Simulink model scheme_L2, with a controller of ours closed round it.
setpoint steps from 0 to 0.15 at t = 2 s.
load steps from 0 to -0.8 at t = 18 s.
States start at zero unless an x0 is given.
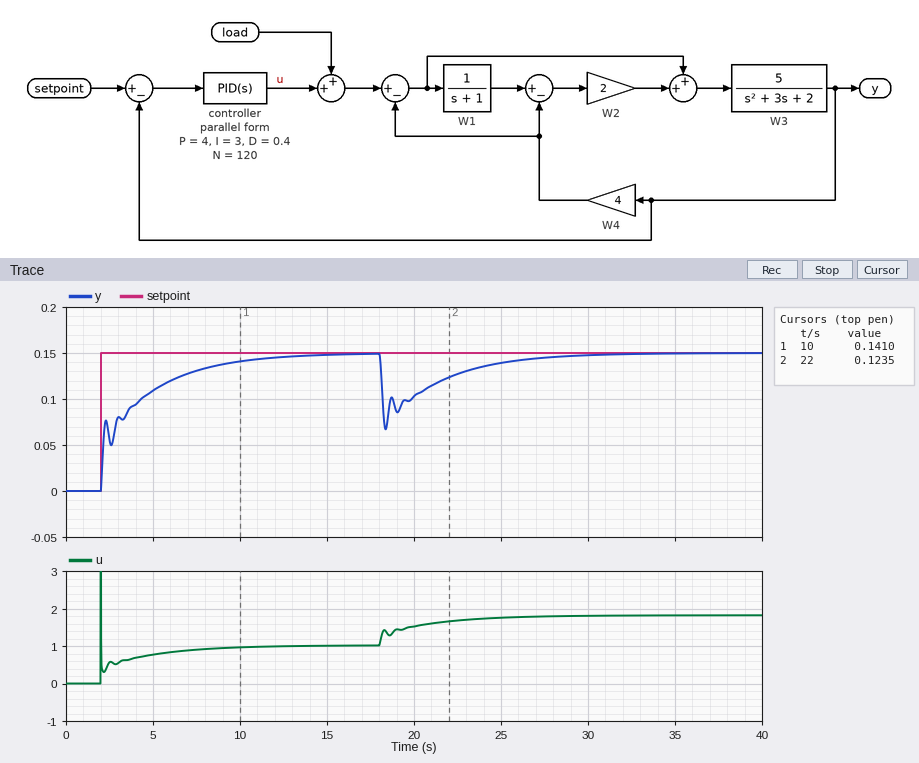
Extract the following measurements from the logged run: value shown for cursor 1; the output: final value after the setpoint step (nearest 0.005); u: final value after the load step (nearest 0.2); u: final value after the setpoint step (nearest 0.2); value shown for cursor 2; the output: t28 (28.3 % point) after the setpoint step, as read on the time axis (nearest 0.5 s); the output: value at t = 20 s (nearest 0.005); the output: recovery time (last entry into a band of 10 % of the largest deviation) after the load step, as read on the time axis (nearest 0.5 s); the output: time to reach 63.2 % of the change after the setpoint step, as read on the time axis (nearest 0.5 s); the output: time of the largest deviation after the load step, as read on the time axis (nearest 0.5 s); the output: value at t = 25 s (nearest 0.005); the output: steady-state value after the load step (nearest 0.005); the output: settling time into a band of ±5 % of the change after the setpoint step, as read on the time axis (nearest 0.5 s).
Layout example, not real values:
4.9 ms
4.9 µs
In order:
0.1410
0.150
1.8
1.0
0.1235
2.0 s
0.105
26.0 s
4.0 s
18.5 s
0.140
0.150
10.5 s
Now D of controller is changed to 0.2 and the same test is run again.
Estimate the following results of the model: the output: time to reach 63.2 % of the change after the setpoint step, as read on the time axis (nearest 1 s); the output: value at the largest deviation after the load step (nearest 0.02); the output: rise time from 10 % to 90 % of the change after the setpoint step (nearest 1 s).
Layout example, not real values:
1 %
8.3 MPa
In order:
4 s
0.06
6 s
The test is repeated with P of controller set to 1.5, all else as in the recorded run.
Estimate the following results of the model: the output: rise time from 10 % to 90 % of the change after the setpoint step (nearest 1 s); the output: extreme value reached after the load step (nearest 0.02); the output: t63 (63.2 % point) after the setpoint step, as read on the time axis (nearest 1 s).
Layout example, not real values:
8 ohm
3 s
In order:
5 s
0.06
4 s
